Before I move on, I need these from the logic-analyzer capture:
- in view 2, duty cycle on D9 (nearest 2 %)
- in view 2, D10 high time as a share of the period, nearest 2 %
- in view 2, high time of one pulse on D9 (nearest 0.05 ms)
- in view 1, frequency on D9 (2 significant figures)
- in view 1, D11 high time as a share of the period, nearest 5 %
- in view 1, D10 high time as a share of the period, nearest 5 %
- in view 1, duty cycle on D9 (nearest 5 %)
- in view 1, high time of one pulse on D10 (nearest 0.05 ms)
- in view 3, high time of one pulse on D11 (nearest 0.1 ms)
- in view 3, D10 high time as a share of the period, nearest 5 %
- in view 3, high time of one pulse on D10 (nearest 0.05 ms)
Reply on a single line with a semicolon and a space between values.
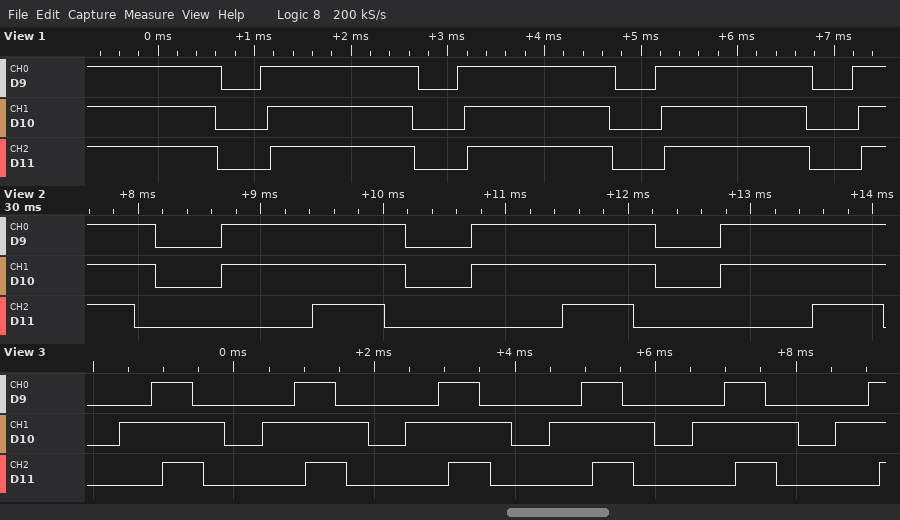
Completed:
74 %; 74 %; 1.50 ms; 490 Hz; 75 %; 75 %; 80 %; 1.50 ms; 0.6 ms; 75 %; 1.50 ms
